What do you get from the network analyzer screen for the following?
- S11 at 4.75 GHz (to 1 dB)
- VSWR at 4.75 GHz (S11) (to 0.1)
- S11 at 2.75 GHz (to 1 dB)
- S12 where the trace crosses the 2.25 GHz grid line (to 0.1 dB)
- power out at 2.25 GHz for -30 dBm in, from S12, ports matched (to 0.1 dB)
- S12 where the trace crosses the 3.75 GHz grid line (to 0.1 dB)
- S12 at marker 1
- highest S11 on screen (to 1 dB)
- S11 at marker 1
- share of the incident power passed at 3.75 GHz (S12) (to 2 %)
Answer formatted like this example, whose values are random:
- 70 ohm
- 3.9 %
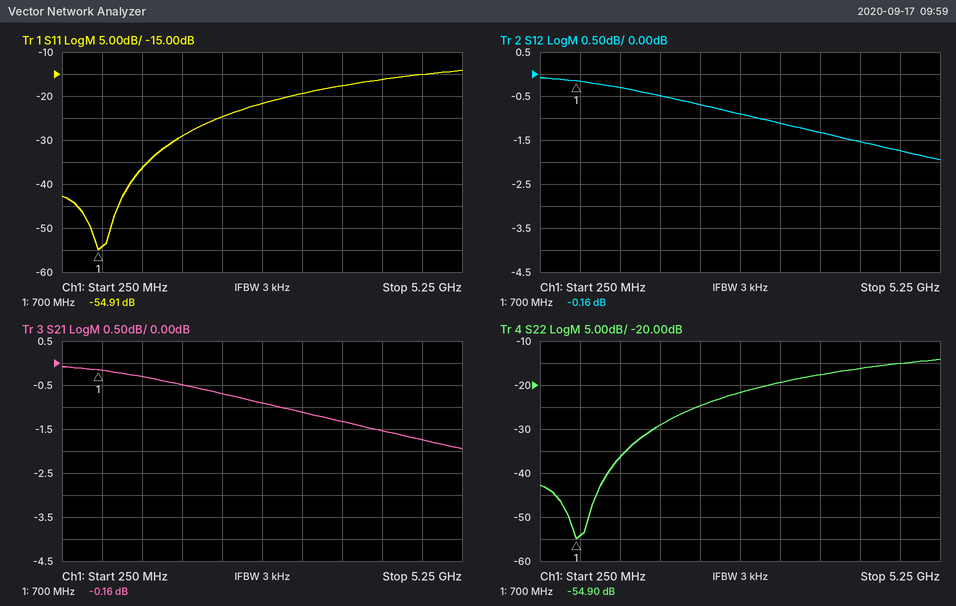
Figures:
- -15 dB
- 1.4
- -22 dB
- -0.7 dB
- -30.7 dBm
- -1.3 dB
- -0.16 dB
- -14 dB
- -54.91 dB
- 74 %
